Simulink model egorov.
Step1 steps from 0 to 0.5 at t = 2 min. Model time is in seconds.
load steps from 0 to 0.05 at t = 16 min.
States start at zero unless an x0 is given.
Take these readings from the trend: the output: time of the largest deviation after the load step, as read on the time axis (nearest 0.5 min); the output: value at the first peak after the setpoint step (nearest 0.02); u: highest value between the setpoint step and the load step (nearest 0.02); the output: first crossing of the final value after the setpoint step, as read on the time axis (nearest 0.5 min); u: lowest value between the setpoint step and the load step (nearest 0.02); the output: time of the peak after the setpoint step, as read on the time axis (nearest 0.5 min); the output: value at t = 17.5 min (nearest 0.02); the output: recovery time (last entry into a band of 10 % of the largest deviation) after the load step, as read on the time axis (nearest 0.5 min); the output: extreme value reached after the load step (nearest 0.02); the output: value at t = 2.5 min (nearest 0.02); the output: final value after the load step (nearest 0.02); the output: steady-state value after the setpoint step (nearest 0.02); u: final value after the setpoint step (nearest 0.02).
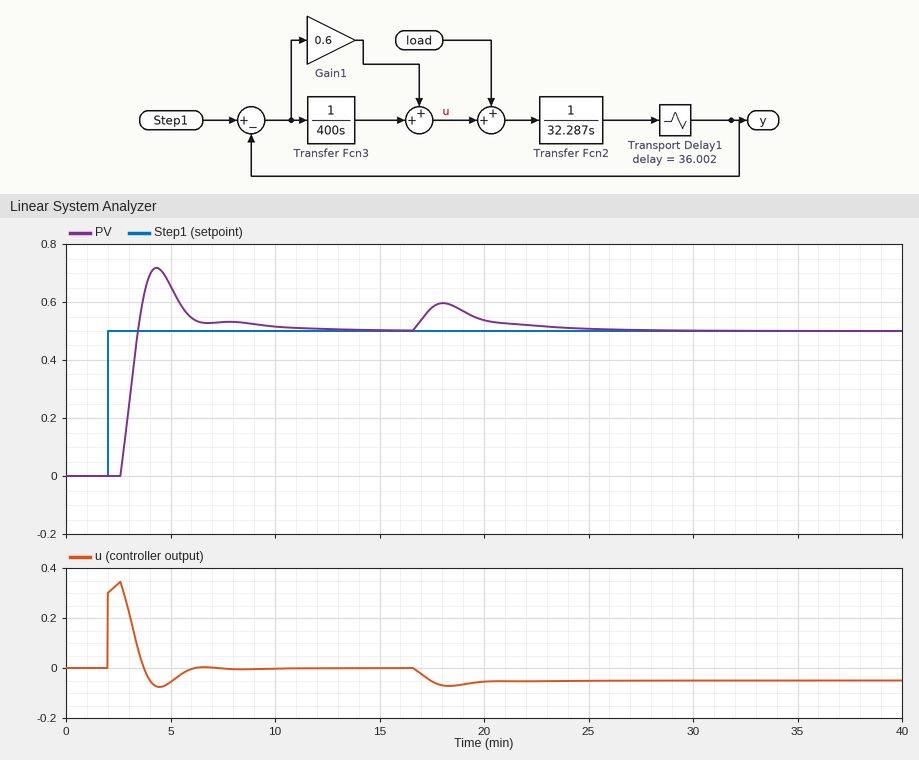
18.0 min
0.72
0.34
3.5 min
-0.08
4.5 min
0.58
24.5 min
0.60
0.00
0.50
0.50
0.00
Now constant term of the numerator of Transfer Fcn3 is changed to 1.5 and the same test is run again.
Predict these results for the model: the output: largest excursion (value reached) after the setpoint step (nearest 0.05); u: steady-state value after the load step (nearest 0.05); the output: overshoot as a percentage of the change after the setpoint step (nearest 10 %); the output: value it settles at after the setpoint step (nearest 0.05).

0.80
-0.05
60 %
0.50
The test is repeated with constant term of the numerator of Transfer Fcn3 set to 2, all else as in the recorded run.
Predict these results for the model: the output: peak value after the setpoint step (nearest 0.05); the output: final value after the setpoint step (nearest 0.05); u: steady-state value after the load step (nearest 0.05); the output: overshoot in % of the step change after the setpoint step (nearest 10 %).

0.85
0.50
-0.05
70 %
